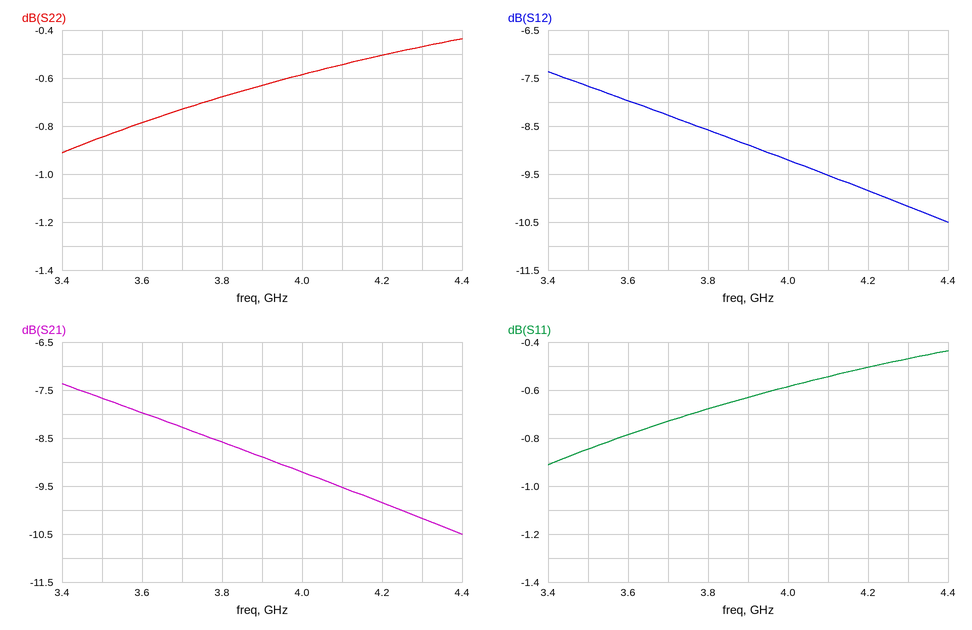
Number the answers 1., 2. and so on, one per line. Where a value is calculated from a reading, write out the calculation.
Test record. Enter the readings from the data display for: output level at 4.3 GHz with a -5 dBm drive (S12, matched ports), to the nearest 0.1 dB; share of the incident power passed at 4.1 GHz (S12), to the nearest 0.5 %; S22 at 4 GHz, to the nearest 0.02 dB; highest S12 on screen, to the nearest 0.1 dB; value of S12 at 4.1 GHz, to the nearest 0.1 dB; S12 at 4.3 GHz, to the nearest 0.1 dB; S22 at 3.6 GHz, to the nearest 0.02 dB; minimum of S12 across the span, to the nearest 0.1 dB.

1. -5 dBm + (-10.2 dB) = -15.2 dBm
2. 10^(-9.5/10) ≈ 11.2 %, so 11.0 % to the nearest 0.5 %
3. -0.58 dB
4. -7.4 dB
5. -9.5 dB
6. -10.2 dB
7. -0.78 dB
8. -10.5 dB
